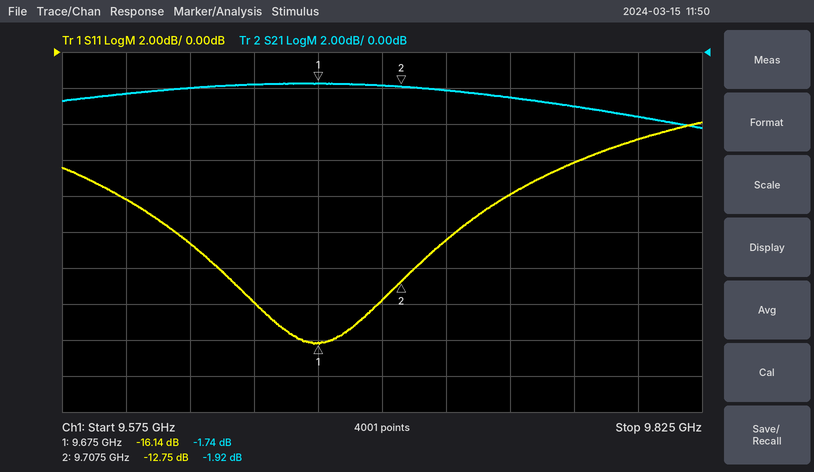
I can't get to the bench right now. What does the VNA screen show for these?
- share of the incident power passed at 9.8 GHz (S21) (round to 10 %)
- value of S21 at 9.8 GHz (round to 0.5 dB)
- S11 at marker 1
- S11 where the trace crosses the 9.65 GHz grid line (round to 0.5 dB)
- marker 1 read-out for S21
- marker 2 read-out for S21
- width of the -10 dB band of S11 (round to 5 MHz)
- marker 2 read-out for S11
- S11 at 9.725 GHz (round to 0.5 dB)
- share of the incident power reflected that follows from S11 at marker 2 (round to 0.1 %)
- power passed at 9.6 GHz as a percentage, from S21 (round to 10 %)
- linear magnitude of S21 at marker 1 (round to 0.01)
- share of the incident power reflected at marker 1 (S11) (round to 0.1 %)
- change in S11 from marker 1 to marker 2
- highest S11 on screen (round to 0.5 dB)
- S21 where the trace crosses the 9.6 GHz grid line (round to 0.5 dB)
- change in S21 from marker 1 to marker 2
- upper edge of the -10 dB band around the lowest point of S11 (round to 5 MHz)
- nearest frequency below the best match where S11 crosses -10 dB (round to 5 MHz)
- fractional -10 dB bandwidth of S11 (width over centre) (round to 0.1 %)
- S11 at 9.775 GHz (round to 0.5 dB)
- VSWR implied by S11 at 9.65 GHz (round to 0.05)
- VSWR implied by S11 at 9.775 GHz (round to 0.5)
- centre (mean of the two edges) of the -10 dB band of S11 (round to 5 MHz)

40 %
-3.5 dB
-16.14 dB
-14.0 dB
-1.74 dB
-1.92 dB
110 MHz
-12.75 dB
-10.5 dB
5.3 %
60 %
0.82
2.4 %
3.39 dB
-4.0 dB
-2.5 dB
-0.18 dB
9.730 GHz
9.620 GHz
1.1 %
-6.0 dB
1.50
3.0
9.675 GHz
